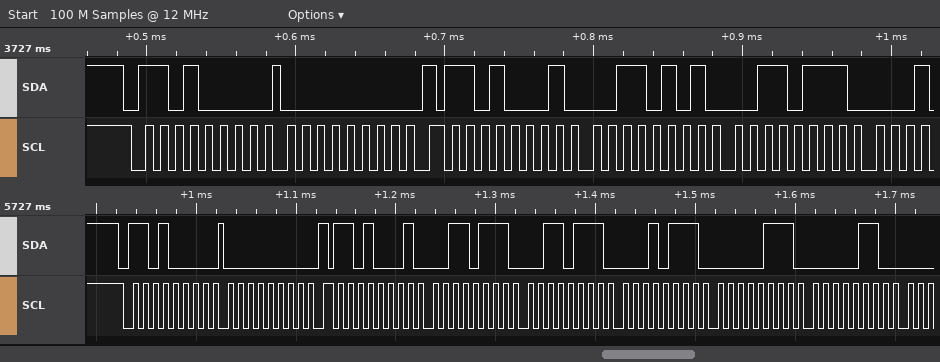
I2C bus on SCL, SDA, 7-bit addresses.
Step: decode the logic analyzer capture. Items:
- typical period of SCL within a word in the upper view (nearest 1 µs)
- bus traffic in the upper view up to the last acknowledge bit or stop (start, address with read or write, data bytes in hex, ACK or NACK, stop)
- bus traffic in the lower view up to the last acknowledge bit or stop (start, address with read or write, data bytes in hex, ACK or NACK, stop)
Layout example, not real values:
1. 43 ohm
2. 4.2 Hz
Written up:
1. 10 µs
2. start, address 68 write ACK, 00 ACK, repeated start, address 68 read ACK, 35 ACK, 37 ACK
3. start, address 68 write ACK, 00 ACK, repeated start, address 68 read ACK, 37 ACK, 37 ACK, 17 ACK, 07 ACK, 06 ACK
